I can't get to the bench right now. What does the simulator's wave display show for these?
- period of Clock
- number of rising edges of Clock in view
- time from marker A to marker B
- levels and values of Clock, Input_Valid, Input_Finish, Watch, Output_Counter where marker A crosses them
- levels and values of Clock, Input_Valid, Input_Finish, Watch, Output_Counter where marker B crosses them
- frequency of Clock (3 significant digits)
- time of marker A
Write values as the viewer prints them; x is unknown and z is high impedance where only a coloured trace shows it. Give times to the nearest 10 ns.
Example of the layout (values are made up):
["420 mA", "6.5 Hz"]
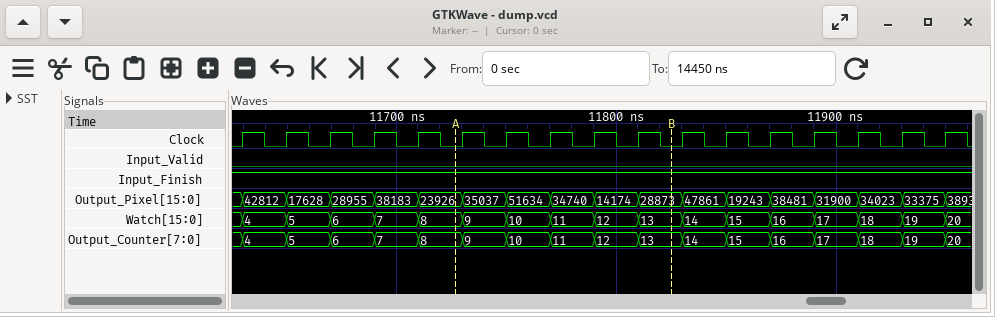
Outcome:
["20 ns", "17", "100 ns", "Clock=0, Input_Valid=0, Input_Finish=1, Watch=8, Output_Counter=8", "Clock=0, Input_Valid=0, Input_Finish=1, Watch=13, Output_Counter=13", "50.0 MHz", "11730 ns"]
